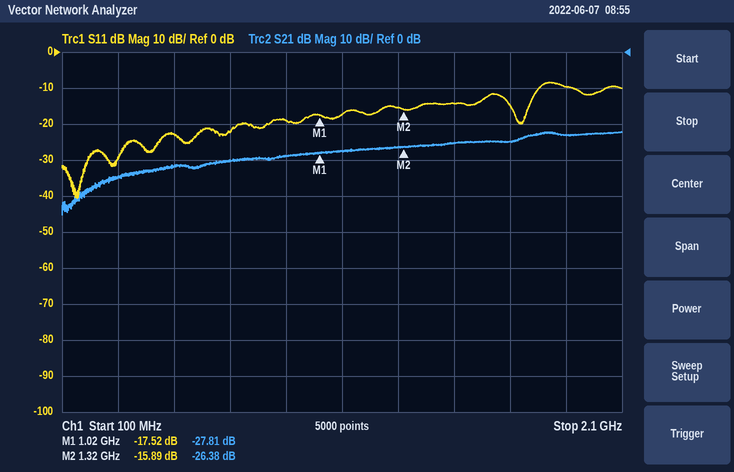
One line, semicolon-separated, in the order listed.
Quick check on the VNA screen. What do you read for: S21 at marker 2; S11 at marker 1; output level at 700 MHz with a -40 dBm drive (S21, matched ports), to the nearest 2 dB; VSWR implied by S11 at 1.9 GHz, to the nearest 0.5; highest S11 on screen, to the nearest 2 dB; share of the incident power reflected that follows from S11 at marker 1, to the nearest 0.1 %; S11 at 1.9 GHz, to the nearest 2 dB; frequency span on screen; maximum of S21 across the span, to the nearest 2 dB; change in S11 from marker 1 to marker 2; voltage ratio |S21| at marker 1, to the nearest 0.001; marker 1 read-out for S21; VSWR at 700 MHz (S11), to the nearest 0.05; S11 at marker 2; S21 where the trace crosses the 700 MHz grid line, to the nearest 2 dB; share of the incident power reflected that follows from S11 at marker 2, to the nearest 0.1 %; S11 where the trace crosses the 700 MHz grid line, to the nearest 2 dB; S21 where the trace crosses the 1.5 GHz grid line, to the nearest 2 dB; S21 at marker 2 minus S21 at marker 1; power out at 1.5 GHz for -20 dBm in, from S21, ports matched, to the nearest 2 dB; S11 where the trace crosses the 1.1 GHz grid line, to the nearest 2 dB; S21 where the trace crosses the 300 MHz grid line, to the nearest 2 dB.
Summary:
-26.38 dB; -17.52 dB; -70 dBm; 2.0; -8 dB; 1.8 %; -10 dB; 2 GHz; -22 dB; 1.63 dB; 0.041; -27.81 dB; 1.15; -15.89 dB; -30 dB; 2.6 %; -22 dB; -26 dB; 1.43 dB; -46 dBm; -18 dB; -34 dB
